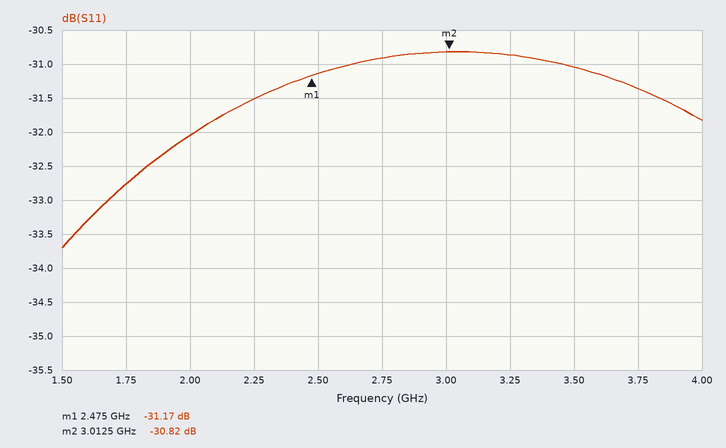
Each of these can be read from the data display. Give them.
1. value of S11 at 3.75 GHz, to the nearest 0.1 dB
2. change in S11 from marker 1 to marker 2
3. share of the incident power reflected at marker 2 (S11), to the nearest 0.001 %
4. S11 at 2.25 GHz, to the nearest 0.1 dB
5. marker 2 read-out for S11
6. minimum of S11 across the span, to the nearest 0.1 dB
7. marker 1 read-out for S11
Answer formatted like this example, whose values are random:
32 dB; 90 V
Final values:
-31.4 dB; 0.35 dB; 0.083 %; -31.5 dB; -30.82 dB; -33.7 dB; -31.17 dB
